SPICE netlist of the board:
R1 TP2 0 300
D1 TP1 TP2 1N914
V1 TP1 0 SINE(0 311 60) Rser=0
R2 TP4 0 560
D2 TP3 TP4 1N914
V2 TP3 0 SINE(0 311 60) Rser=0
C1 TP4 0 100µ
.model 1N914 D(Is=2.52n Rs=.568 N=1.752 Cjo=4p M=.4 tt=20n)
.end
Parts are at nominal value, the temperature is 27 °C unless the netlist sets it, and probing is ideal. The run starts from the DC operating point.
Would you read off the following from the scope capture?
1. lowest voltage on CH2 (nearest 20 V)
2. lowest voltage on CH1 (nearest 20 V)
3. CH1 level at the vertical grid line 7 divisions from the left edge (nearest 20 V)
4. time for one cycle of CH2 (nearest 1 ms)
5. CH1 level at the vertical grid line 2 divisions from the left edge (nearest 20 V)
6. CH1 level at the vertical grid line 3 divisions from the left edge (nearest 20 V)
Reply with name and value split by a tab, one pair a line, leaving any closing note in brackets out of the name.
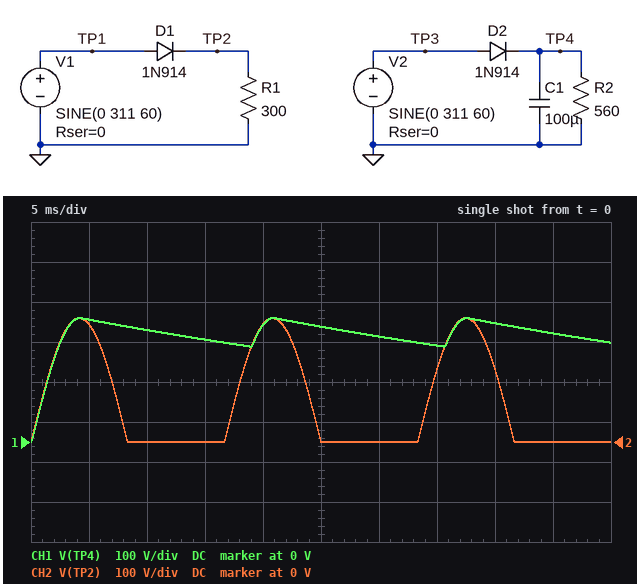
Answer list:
lowest voltage on CH2	0 V
lowest voltage on CH1	0 V
CH1 level at the vertical grid line 7 divisions from the left edge	240 V
time for one cycle of CH2	17 ms
CH1 level at the vertical grid line 2 divisions from the left edge	280 V
CH1 level at the vertical grid line 3 divisions from the left edge	260 V
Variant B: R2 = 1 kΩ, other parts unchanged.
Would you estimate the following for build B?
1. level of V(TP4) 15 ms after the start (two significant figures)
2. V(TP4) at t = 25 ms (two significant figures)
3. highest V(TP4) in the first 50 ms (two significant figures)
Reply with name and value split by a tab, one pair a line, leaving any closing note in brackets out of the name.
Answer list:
level of V(TP4) 15 ms after the start	280 V
V(TP4) at t = 25 ms	300 V
highest V(TP4) in the first 50 ms	310 V
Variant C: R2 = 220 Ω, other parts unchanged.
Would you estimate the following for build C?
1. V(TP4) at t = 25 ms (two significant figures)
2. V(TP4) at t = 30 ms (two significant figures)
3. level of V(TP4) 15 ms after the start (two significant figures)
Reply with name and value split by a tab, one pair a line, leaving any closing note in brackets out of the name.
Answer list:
V(TP4) at t = 25 ms	260 V
V(TP4) at t = 30 ms	210 V
level of V(TP4) 15 ms after the start	190 V
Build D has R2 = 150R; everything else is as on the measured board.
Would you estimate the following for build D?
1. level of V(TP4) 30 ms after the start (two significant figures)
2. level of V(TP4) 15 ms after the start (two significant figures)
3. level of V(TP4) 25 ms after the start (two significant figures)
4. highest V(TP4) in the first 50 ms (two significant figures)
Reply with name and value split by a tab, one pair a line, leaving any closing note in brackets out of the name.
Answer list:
level of V(TP4) 30 ms after the start	170 V
level of V(TP4) 15 ms after the start	150 V
level of V(TP4) 25 ms after the start	240 V
highest V(TP4) in the first 50 ms	310 V
